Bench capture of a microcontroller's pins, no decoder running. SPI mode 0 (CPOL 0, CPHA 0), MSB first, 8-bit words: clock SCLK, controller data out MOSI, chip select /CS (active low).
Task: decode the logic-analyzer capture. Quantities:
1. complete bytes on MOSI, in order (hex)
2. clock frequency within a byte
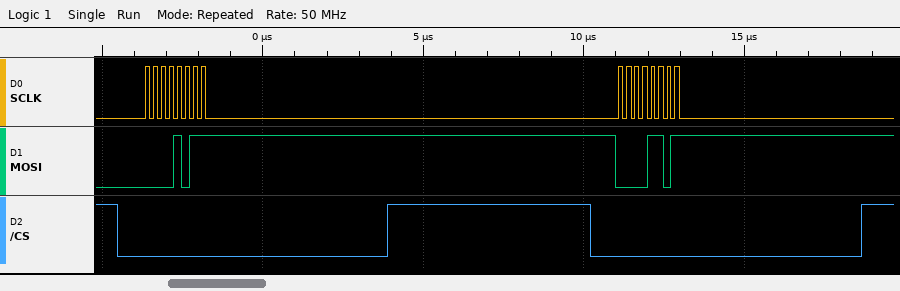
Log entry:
0B 0D
4 MHz
